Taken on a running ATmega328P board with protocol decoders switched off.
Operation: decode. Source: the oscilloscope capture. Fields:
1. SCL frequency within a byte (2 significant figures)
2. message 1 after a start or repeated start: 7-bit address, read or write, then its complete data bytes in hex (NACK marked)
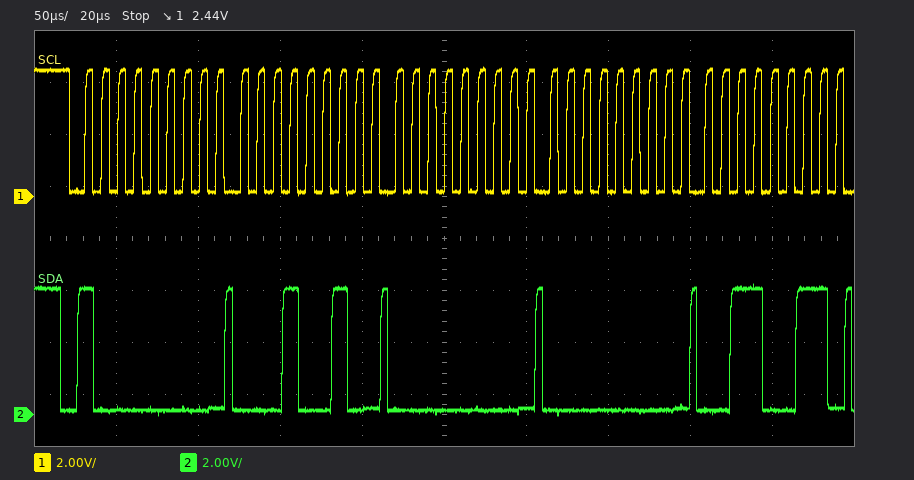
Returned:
100 kHz
0x40 write: 12 00 00 33
